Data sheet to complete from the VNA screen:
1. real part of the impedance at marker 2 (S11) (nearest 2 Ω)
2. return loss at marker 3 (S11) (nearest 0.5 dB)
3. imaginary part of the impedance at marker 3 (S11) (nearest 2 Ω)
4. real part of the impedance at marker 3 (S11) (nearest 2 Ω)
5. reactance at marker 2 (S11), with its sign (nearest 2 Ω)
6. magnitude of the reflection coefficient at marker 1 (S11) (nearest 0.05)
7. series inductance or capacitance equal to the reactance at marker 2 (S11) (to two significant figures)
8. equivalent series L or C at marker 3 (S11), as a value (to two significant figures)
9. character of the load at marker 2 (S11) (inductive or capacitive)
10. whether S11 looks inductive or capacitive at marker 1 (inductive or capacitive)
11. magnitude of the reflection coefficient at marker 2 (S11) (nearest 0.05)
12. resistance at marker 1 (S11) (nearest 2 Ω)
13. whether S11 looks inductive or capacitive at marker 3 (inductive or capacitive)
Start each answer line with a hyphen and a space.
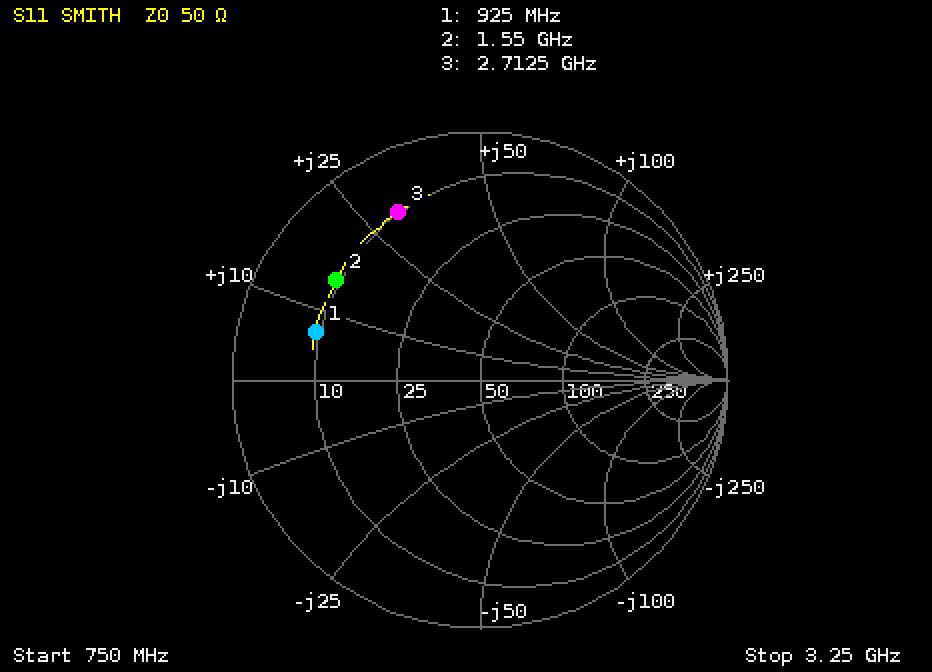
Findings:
- 10 Ω
- 2.5 dB
- +30 Ω
- 10 Ω
- +16 Ω
- 0.70
- 1.6 nH
- 1.8 nH
- inductive
- inductive
- 0.70
- 10 Ω
- inductive
